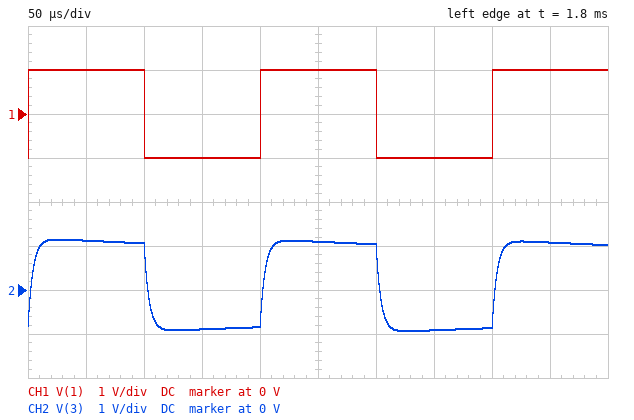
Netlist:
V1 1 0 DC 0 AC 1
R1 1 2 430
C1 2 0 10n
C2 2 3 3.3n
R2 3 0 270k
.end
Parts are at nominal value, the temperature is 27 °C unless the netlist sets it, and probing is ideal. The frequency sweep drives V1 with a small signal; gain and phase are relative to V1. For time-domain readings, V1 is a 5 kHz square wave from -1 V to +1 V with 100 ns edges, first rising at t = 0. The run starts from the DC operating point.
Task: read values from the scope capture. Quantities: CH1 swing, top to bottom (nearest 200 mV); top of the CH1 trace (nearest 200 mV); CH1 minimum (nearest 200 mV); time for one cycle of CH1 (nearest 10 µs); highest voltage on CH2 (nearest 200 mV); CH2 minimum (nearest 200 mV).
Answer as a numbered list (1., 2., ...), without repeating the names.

1. 2.0 V
2. 1.0 V
3. -1.0 V
4. 200 µs
5. 1.2 V
6. -1.0 V
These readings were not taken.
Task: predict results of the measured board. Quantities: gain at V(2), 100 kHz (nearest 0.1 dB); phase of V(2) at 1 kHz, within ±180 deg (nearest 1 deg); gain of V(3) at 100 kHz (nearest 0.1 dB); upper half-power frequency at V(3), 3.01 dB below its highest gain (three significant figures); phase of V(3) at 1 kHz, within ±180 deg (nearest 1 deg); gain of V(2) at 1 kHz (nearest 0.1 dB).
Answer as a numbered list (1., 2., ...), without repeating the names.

1. -9.2 dB
2. -2 deg
3. -9.2 dB
4. 37.4 kHz
5. 9 deg
6. 0 dB
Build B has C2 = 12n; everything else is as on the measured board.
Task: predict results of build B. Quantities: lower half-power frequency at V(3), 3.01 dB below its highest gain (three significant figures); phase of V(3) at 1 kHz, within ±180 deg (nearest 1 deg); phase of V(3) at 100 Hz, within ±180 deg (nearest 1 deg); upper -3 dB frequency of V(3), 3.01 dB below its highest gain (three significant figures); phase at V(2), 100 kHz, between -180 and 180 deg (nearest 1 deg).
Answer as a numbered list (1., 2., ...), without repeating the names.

1. 48.9 Hz
2. 1 deg
3. 26 deg
4. 37.2 kHz
5. -70 deg
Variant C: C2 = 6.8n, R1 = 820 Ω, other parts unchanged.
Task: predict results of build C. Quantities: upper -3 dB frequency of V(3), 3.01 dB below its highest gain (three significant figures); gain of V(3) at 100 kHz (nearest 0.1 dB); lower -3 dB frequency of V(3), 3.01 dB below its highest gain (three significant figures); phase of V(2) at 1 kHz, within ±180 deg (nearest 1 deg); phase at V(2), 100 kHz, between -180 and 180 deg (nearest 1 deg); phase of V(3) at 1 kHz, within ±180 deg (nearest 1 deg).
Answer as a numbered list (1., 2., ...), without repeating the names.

1. 19.6 kHz
2. -14.4 dB
3. 85.7 Hz
4. -3 deg
5. -79 deg
6. 2 deg
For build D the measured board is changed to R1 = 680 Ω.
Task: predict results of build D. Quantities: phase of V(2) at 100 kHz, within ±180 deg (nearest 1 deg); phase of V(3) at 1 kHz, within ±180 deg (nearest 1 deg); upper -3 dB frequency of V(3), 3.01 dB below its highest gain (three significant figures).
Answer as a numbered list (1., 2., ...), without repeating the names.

1. -77 deg
2. 8 deg
3. 23.8 kHz
